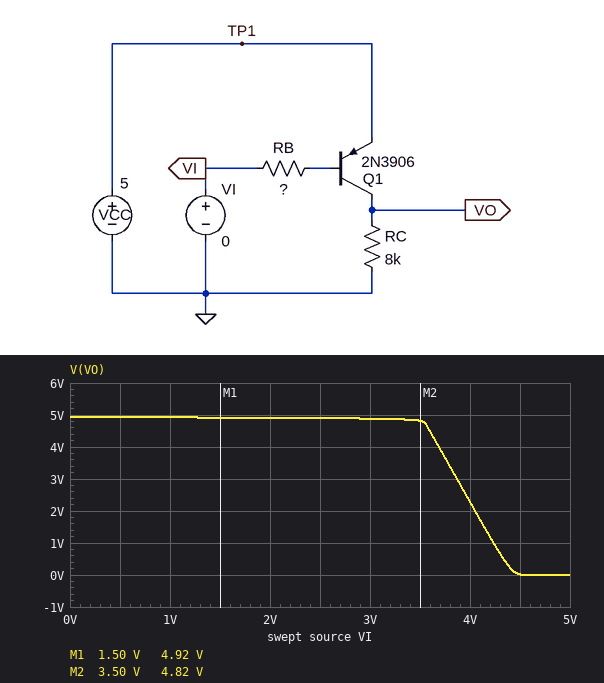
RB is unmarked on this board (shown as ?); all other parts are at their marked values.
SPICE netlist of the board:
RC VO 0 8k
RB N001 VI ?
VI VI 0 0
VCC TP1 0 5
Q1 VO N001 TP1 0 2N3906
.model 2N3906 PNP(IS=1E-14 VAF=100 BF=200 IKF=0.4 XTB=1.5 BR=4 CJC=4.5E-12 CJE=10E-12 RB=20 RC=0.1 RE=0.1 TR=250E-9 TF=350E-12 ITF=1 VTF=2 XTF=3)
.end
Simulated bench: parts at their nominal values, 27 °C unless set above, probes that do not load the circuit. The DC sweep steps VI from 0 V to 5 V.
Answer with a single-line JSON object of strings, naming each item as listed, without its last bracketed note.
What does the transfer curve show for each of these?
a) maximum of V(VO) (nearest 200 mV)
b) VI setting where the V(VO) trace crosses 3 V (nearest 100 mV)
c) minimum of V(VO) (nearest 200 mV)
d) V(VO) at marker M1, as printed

{"maximum of V(VO)": "5.0 V", "VI setting where the V(VO) trace crosses 3 V": "3.9 V", "minimum of V(VO)": "0 V", "V(VO) at marker M1, as printed": "4.92 V"}
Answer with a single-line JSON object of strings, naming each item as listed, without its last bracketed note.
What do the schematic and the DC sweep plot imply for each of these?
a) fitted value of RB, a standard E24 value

{"fitted value of RB, a standard E24 value": "270 kΩ"}
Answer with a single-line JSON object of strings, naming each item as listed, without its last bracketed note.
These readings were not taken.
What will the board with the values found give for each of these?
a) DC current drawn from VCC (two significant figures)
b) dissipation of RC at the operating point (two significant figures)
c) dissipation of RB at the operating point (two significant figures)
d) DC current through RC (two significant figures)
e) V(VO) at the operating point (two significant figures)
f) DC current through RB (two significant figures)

{"DC current drawn from VCC": "630 µA", "dissipation of RC at the operating point": "3.0 mW", "dissipation of RB at the operating point": "70 µW", "DC current through RC": "620 µA", "V(VO) at the operating point": "4.9 V", "DC current through RB": "16 µA"}
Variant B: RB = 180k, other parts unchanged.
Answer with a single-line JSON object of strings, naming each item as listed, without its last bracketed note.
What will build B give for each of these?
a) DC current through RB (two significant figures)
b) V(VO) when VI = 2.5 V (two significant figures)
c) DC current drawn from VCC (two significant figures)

{"DC current through RB": "24 µA", "V(VO) when VI = 2.5 V": "4.9 V", "DC current drawn from VCC": "640 µA"}
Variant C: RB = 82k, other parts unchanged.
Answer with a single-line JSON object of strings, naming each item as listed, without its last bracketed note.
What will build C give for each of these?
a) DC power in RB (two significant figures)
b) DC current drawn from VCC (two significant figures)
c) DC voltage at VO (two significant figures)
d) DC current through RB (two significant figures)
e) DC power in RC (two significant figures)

{"DC power in RB": "230 µW", "DC current drawn from VCC": "670 µA", "DC voltage at VO": "5.0 V", "DC current through RB": "53 µA", "DC power in RC": "3.1 mW"}
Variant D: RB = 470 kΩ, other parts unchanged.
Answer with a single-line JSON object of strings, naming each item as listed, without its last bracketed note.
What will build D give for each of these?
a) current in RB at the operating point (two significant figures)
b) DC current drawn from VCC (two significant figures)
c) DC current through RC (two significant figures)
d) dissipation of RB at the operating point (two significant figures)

{"current in RB at the operating point": "9.3 µA", "DC current drawn from VCC": "620 µA", "DC current through RC": "610 µA", "dissipation of RB at the operating point": "40 µW"}
